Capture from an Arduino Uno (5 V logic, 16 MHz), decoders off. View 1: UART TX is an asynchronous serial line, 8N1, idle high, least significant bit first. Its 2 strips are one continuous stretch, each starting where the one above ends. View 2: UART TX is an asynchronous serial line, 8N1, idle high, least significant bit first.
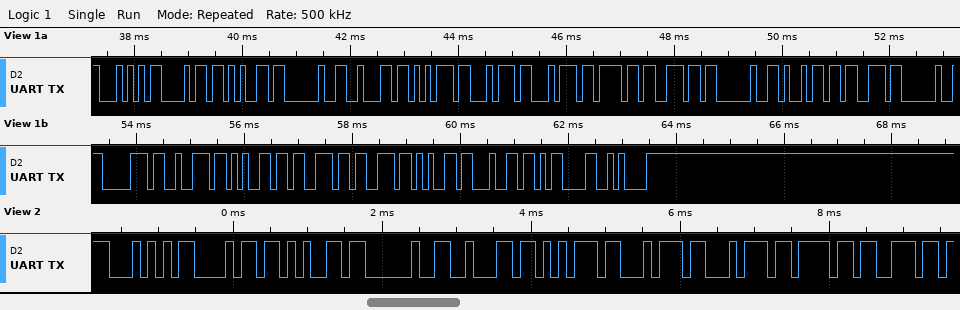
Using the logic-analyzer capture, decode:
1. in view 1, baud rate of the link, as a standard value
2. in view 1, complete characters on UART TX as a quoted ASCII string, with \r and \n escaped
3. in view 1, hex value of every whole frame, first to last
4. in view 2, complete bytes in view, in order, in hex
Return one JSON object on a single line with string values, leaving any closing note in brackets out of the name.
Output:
{"in view 1, baud rate of the link, as a standard value": "9600 baud", "in view 1, complete characters on UART TX as a quoted ASCII string, with \\r and \\n escaped": "\"The button is pressed\\r\\n\"", "in view 1, hex value of every whole frame, first to last": "54 68 65 20 62 75 74 74 6F 6E 20 69 73 20 70 72 65 73 73 65 64 0D 0A", "in view 2, complete bytes in view, in order, in hex": "54 68 65 20 62 75 74 74 6F 6E"}
